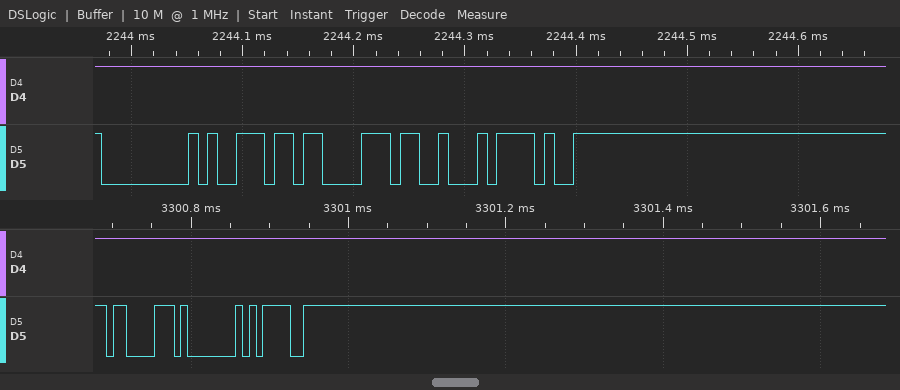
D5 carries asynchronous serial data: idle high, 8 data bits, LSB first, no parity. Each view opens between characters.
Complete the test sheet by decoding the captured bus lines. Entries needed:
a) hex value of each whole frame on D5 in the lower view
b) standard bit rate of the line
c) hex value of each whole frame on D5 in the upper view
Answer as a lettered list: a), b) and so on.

a) C3, 01, 3D
b) 115200 baud
c) 00, B9, C3, 13, 2F
